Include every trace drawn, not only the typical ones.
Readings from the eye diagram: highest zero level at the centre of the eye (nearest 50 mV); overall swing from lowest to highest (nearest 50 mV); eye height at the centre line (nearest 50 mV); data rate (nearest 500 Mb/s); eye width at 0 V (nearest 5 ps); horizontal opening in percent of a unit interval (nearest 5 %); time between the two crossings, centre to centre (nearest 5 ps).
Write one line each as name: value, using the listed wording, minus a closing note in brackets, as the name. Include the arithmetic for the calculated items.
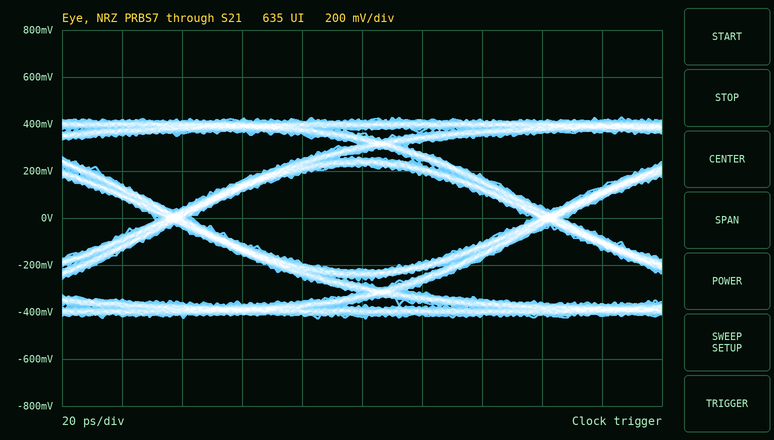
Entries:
highest zero level at the centre of the eye: -200 mV
overall swing from lowest to highest: 850 mV
eye height at the centre line: 450 mV
data rate: 8.0 Gb/s
eye width at 0 V: 115 ps
horizontal opening in percent of a unit interval: 115 ps / 125 ps ≈ 92.0 %, so 90 % to the nearest 5 %
time between the two crossings, centre to centre: 125 ps
